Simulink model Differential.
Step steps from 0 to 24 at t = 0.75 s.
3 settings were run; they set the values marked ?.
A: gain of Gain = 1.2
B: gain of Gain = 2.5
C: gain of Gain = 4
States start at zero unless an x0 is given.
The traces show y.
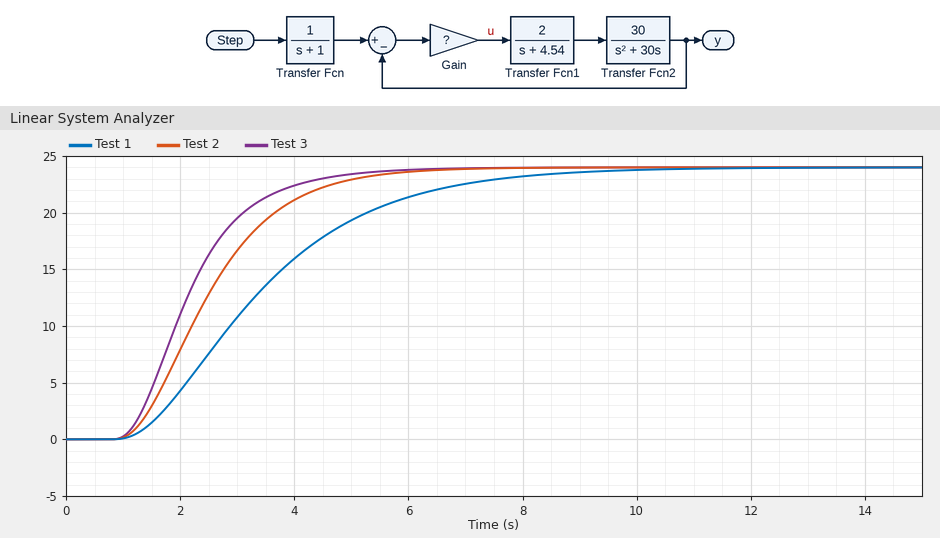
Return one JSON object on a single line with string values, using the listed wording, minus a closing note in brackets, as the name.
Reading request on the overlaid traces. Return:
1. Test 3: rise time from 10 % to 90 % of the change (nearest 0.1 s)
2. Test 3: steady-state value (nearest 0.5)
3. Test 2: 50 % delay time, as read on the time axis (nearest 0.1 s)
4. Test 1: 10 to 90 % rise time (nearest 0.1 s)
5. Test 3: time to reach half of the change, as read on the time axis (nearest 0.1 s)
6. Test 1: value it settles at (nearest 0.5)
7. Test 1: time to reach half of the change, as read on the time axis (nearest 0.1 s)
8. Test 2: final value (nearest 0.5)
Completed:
{"Test 3: rise time from 10 % to 90 % of the change": "2.3 s", "Test 3: steady-state value": "24.0", "Test 2: 50 % delay time, as read on the time axis": "2.4 s", "Test 1: 10 to 90 % rise time": "4.5 s", "Test 3: time to reach half of the change, as read on the time axis": "2.1 s", "Test 1: value it settles at": "24.0", "Test 1: time to reach half of the change, as read on the time axis": "3.2 s", "Test 2: final value": "24.0"}
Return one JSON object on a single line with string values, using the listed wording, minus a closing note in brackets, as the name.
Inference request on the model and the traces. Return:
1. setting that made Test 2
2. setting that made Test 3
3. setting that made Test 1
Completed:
{"setting that made Test 2": "B", "setting that made Test 3": "C", "setting that made Test 1": "A"}
